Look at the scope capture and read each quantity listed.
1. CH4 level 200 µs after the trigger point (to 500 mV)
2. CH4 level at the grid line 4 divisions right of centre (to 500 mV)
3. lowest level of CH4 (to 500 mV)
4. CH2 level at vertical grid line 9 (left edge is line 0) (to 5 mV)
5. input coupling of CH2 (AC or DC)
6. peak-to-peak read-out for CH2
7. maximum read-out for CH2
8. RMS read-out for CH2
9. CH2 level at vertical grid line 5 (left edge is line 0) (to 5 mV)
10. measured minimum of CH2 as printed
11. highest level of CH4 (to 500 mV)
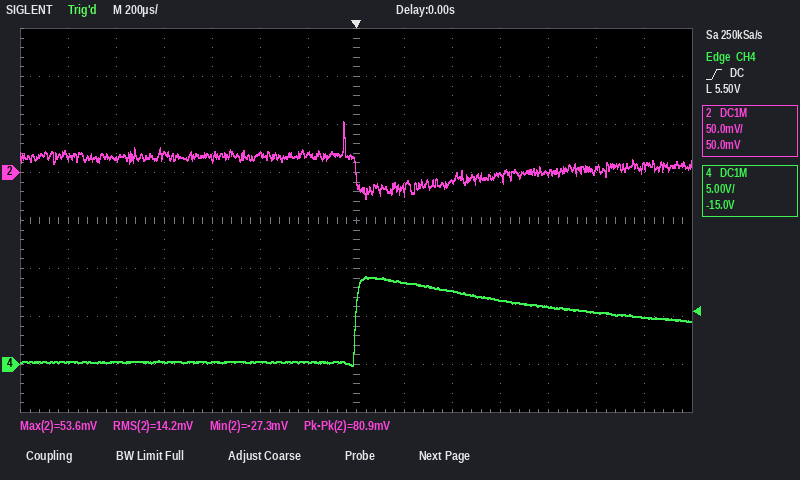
8.5 V
6.0 V
0.0 V
-10 mV
DC
80.9 mV
53.6 mV
14.2 mV
20 mV
-27.3 mV
9.0 V
